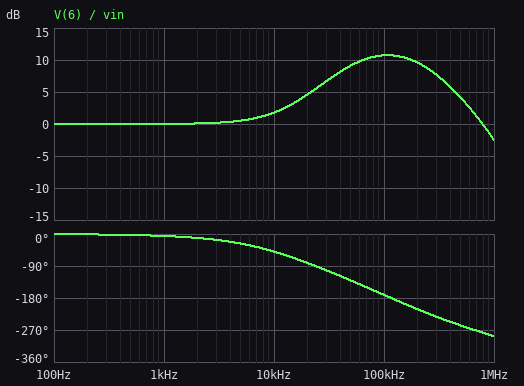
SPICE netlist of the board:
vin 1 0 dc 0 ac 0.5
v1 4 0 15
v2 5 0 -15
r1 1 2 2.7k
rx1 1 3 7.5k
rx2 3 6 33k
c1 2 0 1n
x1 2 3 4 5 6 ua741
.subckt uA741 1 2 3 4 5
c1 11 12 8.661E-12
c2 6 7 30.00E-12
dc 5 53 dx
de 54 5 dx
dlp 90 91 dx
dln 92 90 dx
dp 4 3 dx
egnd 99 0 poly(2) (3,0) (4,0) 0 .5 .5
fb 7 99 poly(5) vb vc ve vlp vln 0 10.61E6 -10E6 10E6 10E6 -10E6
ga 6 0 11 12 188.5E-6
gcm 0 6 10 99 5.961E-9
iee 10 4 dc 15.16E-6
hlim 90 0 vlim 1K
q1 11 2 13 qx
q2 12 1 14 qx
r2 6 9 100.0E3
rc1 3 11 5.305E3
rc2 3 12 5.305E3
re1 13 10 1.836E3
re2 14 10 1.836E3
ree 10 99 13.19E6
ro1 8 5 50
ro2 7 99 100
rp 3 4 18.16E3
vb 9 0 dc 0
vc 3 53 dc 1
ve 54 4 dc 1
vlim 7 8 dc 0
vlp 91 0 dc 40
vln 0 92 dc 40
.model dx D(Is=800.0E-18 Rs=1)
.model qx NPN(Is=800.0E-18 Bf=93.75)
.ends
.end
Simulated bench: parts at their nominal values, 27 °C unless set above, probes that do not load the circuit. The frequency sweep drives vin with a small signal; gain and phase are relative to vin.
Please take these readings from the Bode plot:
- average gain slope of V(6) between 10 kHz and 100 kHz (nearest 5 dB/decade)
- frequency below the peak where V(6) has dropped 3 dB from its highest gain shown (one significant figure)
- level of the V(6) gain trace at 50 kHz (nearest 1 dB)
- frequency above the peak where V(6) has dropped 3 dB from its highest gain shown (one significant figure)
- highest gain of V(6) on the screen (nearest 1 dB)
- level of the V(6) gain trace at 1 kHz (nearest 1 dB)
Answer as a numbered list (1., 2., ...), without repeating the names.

1. 10 dB/decade
2. 40 kHz
3. 9 dB
4. 300 kHz
5. 11 dB
6. 0 dB
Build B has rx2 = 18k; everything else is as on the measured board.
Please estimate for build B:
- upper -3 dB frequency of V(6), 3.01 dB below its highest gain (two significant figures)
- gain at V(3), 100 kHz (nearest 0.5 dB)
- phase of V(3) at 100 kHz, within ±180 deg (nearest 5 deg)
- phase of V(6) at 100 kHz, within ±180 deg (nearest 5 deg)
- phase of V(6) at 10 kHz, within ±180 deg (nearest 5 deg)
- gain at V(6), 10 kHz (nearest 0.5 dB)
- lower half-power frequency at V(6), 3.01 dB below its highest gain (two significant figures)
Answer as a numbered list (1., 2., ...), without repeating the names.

1. 430 kHz
2. -10.5 dB
3. -60 deg
4. -155 deg
5. -35 deg
6. 0.5 dB
7. 34 kHz
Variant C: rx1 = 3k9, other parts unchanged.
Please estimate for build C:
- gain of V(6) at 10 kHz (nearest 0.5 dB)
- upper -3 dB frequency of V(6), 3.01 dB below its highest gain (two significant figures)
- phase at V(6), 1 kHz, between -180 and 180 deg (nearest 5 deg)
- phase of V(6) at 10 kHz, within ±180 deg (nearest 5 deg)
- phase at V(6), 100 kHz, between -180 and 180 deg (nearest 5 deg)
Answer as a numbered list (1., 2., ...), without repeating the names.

1. 4.5 dB
2. 200 kHz
3. -10 deg
4. -70 deg
5. 170 deg
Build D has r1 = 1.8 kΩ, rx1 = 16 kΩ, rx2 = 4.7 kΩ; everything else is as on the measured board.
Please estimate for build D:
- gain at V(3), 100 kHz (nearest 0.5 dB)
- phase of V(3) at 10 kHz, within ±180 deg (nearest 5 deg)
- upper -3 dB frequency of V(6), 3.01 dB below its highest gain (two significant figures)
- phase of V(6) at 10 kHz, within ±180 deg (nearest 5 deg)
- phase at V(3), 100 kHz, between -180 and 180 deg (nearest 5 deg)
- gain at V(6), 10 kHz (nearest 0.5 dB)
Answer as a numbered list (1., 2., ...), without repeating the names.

1. -4.0 dB
2. -5 deg
3. 97 kHz
4. -10 deg
5. -55 deg
6. 0 dB
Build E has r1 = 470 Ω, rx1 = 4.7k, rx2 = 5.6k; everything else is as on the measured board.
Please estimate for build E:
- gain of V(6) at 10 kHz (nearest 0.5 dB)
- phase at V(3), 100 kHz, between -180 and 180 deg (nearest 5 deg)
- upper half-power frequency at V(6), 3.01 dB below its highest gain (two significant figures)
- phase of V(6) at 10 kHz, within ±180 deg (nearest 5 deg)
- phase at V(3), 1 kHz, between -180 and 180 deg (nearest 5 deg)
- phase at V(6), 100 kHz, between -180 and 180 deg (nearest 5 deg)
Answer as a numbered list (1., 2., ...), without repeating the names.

1. 0 dB
2. -20 deg
3. 720 kHz
4. -5 deg
5. 0 deg
6. -50 deg
